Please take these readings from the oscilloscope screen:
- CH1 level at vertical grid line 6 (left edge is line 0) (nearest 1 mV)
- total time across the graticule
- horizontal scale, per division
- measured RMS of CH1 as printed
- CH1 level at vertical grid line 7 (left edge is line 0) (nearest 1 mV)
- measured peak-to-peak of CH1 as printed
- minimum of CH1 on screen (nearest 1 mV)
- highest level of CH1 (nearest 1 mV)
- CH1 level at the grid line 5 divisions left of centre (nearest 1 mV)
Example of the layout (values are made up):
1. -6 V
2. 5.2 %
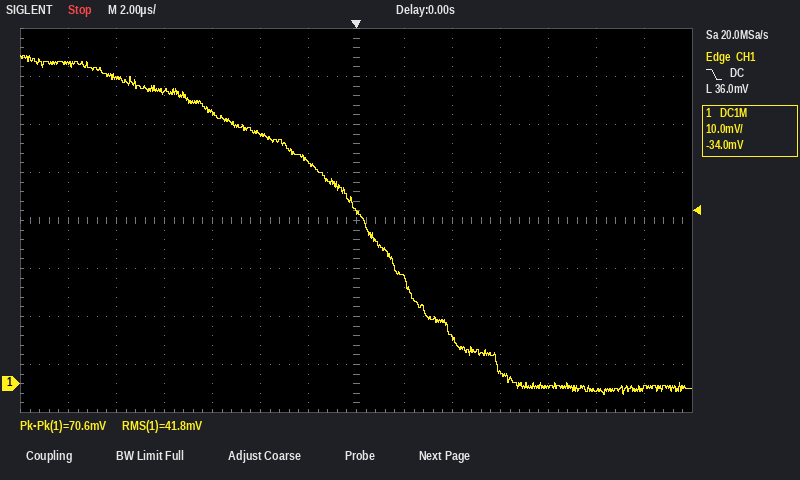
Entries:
1. 46 mV
2. 28 µs
3. 2 µs
4. 41.8 mV
5. 36 mV
6. 70.6 mV
7. -2 mV
8. 68 mV
9. 64 mV
